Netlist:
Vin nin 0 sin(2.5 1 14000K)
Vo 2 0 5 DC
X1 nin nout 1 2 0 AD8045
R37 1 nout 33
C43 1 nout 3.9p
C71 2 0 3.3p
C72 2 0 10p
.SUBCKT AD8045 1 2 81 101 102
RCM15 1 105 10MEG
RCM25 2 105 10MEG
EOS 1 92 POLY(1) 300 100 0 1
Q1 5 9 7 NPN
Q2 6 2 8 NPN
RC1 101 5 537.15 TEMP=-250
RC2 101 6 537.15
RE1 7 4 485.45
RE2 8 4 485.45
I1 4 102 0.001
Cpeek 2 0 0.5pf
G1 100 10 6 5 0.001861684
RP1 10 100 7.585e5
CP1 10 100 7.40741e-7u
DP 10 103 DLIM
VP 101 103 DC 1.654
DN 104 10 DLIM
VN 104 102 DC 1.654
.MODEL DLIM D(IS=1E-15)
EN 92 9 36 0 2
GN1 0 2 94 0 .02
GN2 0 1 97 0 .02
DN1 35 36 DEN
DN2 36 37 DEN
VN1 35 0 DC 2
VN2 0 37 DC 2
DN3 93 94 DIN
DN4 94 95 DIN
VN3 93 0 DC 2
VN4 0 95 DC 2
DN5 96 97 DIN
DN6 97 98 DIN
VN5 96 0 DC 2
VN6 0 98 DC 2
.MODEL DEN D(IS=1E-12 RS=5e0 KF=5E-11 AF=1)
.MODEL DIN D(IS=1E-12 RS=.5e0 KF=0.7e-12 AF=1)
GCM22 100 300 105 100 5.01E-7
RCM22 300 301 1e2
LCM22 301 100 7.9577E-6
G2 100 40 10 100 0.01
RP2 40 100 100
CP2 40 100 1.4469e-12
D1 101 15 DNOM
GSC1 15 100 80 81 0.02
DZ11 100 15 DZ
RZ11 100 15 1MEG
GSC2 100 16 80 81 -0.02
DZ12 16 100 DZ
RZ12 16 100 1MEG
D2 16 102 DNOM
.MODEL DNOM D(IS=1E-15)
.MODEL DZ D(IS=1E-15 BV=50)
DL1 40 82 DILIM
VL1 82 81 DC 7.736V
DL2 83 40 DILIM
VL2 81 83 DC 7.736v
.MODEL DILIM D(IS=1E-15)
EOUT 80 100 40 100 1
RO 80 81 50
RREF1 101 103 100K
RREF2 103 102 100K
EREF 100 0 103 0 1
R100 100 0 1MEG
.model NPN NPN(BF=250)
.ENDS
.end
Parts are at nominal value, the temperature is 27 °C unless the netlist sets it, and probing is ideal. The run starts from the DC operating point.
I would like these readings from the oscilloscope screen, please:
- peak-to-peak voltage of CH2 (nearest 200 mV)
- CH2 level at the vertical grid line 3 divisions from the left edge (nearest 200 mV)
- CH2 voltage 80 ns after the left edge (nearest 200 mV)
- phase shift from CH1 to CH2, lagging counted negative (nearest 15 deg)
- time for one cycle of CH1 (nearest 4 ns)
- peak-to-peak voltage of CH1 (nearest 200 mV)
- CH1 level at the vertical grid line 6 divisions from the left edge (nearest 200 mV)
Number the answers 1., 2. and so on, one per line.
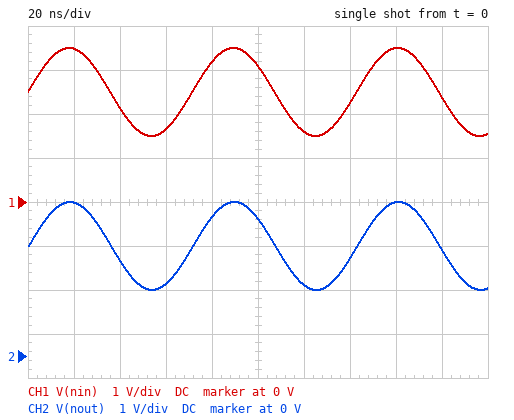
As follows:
1. 2.0 V
2. 1.6 V
3. 3.2 V
4. 0 deg
5. 72 ns
6. 2.0 V
7. 1.6 V
